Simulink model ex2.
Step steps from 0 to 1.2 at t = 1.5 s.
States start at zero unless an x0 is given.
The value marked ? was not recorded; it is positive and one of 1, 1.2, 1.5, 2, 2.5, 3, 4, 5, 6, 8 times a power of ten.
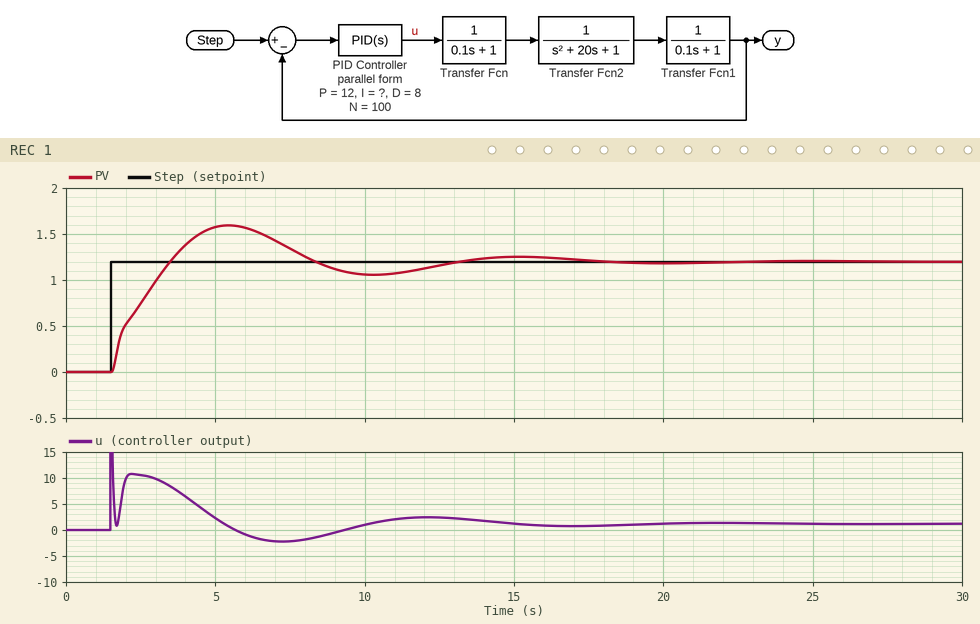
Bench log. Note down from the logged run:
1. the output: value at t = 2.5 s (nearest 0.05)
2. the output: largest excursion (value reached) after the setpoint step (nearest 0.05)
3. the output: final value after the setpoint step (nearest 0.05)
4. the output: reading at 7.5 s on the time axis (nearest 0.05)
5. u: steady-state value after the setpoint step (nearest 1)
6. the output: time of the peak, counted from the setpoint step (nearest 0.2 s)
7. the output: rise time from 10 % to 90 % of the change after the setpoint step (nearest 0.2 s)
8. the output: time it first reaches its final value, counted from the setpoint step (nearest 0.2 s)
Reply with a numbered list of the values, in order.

1. 0.75
2. 1.60
3. 1.20
4. 1.35
5. 1
6. 4.0 s
7. 1.6 s
8. 2.0 s
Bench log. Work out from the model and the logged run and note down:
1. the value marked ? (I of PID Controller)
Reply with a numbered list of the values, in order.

1. 12
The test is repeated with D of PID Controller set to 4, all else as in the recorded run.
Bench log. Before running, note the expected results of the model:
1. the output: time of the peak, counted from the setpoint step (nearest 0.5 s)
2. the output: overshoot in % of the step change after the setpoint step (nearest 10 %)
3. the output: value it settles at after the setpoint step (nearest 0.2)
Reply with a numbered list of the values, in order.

1. 3.5 s
2. 40 %
3. 1.2
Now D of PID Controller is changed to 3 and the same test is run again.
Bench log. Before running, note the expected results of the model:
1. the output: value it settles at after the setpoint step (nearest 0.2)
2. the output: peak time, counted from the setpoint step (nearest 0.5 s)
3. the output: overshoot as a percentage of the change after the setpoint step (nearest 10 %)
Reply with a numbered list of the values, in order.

1. 1.2
2. 3.5 s
3. 40 %
